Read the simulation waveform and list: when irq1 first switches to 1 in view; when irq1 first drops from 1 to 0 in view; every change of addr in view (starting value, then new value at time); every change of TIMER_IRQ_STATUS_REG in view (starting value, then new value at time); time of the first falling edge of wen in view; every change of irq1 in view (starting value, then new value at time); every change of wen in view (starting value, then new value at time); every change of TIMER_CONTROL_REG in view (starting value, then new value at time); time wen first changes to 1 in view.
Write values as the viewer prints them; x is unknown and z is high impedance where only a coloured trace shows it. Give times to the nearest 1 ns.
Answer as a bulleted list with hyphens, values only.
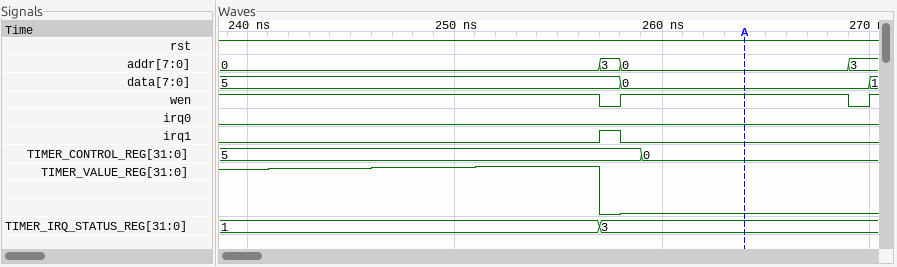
- 257 ns
- 258 ns
- 0, 3 at 257 ns, 0 at 258 ns, 3 at 269 ns
- 1, 3 at 257 ns
- 257 ns
- 0, 1 at 257 ns, 0 at 258 ns
- 1, 0 at 257 ns, 1 at 258 ns, 0 at 269 ns, 1 at 270 ns
- 5, 0 at 259 ns
- 258 ns
